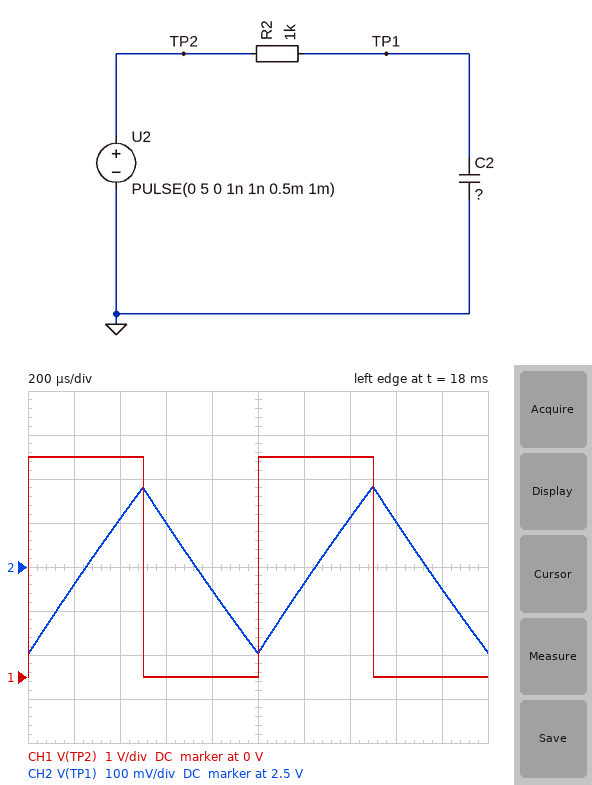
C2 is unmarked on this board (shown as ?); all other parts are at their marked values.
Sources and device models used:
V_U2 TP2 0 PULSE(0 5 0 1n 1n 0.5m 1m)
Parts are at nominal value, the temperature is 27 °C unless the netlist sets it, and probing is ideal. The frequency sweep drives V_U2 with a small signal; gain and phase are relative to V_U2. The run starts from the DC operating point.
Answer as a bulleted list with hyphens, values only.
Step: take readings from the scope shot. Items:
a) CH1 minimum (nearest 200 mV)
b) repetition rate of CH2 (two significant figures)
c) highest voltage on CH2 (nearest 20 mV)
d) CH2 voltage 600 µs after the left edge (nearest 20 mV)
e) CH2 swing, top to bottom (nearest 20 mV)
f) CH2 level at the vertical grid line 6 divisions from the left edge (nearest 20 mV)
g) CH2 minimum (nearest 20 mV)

- 0 V
- 1.0 kHz
- 2.68 V
- 2.60 V
- 380 mV
- 2.46 V
- 2.30 V
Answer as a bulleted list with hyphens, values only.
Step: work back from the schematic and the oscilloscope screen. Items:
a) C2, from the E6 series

- 3.3 µF
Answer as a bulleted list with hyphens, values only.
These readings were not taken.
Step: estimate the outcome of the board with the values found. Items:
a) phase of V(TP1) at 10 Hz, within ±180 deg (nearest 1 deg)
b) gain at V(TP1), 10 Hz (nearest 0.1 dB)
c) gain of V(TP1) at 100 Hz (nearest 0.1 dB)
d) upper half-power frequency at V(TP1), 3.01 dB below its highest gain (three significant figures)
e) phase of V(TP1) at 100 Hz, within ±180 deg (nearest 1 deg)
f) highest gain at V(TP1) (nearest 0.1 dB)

- -12 deg
- -0.2 dB
- -7.2 dB
- 48.2 Hz
- -64 deg
- 0 dB
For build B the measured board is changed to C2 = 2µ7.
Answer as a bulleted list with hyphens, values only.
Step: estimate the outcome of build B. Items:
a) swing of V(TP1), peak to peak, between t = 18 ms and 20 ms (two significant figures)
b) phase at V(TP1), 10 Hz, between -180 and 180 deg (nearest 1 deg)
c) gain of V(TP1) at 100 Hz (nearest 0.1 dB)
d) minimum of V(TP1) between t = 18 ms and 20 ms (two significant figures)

- 460 mV
- -10 deg
- -5.9 dB
- 2.3 V
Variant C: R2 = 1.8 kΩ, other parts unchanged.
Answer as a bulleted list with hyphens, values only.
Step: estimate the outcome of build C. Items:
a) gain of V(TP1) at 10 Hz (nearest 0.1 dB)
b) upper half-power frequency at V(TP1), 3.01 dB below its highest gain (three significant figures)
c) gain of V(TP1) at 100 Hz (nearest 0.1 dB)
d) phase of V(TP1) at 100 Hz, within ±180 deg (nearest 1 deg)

- -0.6 dB
- 26.8 Hz
- -11.7 dB
- -75 deg
